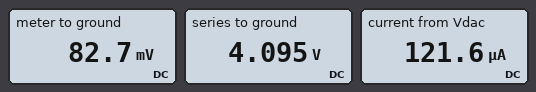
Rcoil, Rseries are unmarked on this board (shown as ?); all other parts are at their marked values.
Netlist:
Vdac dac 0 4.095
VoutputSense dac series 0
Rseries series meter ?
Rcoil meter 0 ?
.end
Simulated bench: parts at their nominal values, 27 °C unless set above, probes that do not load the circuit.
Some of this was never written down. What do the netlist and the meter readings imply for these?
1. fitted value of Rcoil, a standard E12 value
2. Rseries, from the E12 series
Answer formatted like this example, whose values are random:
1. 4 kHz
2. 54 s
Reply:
1. 680 Ω
2. 33 kΩ
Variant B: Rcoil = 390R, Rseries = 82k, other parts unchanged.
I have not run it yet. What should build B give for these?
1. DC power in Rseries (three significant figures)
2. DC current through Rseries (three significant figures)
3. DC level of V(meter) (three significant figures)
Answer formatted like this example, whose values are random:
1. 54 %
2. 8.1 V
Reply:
1. 203 µW
2. 49.7 µA
3. 19.4 mV
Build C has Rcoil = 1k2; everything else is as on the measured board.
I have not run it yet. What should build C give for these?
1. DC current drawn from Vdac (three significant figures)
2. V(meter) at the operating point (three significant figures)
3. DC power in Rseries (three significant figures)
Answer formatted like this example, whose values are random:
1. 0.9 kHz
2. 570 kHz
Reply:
1. 120 µA
2. 144 mV
3. 473 µW
